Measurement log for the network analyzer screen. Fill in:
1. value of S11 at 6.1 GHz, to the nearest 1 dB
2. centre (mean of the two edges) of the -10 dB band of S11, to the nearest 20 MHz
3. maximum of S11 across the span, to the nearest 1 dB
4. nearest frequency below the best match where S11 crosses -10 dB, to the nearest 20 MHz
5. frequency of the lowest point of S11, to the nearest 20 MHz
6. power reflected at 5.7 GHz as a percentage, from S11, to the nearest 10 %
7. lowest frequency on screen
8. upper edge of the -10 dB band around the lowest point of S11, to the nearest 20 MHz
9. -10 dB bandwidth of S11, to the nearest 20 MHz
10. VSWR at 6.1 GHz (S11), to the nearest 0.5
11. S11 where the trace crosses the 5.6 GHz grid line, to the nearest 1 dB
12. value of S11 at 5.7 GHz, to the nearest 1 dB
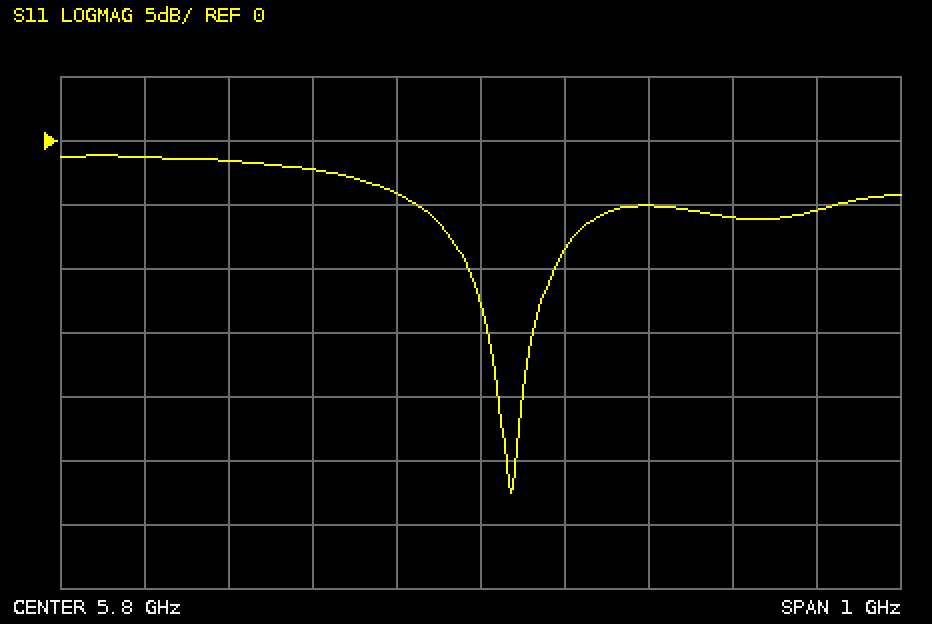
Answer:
-6 dB
5.84 GHz
-1 dB
5.78 GHz
5.84 GHz
40 %
5.3 GHz
5.88 GHz
100 MHz
3.0
-2 dB
-4 dB
